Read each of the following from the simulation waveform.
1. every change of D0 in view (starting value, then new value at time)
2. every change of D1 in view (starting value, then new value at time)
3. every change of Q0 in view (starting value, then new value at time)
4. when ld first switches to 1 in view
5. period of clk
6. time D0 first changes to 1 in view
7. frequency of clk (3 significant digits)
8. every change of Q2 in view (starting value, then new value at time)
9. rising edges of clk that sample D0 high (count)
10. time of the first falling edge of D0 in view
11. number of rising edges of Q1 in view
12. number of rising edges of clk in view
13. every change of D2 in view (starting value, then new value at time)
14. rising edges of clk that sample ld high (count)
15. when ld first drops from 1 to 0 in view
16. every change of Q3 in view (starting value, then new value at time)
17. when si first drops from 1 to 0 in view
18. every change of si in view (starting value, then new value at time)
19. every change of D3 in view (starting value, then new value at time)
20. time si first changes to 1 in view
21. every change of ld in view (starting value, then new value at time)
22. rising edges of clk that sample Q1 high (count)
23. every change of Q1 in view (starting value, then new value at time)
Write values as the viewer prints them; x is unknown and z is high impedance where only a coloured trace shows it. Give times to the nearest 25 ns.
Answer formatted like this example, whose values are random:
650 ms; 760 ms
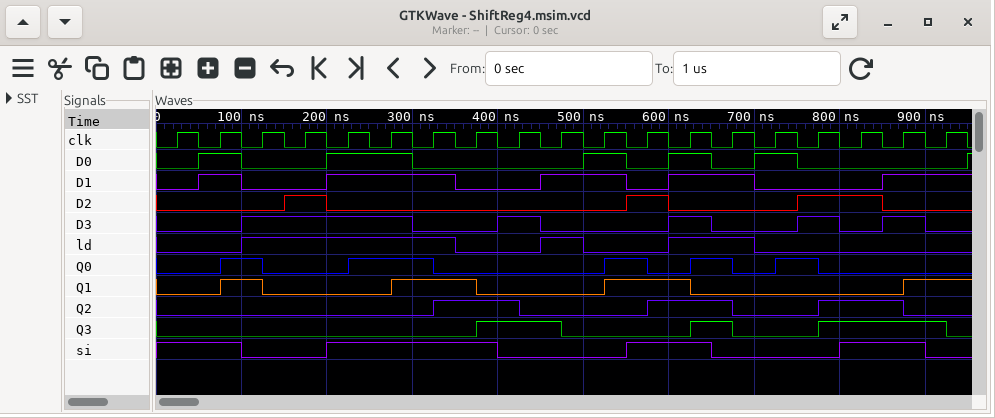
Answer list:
0, 1 at 50 ns, 0 at 100 ns, 1 at 200 ns, 0 at 300 ns, 1 at 500 ns, 0 at 550 ns, 1 at 600 ns, 0 at 650 ns, 1 at 700 ns, 0 at 750 ns, 1 at 950 ns; 0, 1 at 50 ns, 0 at 100 ns, 1 at 200 ns, 0 at 350 ns, 1 at 450 ns, 0 at 550 ns, 1 at 600 ns, 0 at 700 ns, 1 at 850 ns; 0, 1 at 75 ns, 0 at 125 ns, 1 at 225 ns, 0 at 325 ns, 1 at 525 ns, 0 at 575 ns, 1 at 625 ns, 0 at 675 ns, 1 at 725 ns, 0 at 775 ns; 100 ns; 50 ns; 50 ns; 20.0 MHz; 0, 1 at 325 ns, 0 at 425 ns, 1 at 575 ns, 0 at 675 ns, 1 at 775 ns, 0 at 875 ns; 6; 100 ns; 4; 19; 0, 1 at 150 ns, 0 at 200 ns, 1 at 550 ns, 0 at 600 ns, 1 at 750 ns, 0 at 850 ns; 8; 350 ns; 0, 1 at 375 ns, 0 at 475 ns, 1 at 625 ns, 0 at 675 ns, 1 at 775 ns, 0 at 925 ns; 100 ns; 1, 0 at 100 ns, 1 at 200 ns, 0 at 400 ns, 1 at 550 ns, 0 at 650 ns, 1 at 800 ns, 0 at 900 ns; 0, 1 at 100 ns, 0 at 300 ns, 1 at 400 ns, 0 at 450 ns, 1 at 600 ns, 0 at 650 ns, 1 at 750 ns, 0 at 800 ns, 1 at 850 ns, 0 at 900 ns; 200 ns; 0, 1 at 100 ns, 0 at 350 ns, 1 at 450 ns, 0 at 500 ns, 1 at 600 ns, 0 at 700 ns; 6; 0, 1 at 75 ns, 0 at 125 ns, 1 at 275 ns, 0 at 375 ns, 1 at 525 ns, 0 at 625 ns, 1 at 875 ns
